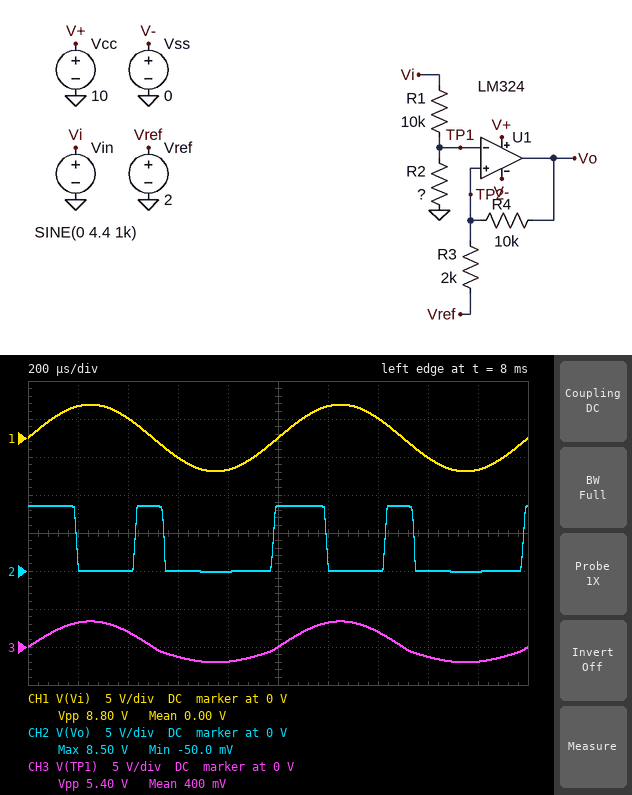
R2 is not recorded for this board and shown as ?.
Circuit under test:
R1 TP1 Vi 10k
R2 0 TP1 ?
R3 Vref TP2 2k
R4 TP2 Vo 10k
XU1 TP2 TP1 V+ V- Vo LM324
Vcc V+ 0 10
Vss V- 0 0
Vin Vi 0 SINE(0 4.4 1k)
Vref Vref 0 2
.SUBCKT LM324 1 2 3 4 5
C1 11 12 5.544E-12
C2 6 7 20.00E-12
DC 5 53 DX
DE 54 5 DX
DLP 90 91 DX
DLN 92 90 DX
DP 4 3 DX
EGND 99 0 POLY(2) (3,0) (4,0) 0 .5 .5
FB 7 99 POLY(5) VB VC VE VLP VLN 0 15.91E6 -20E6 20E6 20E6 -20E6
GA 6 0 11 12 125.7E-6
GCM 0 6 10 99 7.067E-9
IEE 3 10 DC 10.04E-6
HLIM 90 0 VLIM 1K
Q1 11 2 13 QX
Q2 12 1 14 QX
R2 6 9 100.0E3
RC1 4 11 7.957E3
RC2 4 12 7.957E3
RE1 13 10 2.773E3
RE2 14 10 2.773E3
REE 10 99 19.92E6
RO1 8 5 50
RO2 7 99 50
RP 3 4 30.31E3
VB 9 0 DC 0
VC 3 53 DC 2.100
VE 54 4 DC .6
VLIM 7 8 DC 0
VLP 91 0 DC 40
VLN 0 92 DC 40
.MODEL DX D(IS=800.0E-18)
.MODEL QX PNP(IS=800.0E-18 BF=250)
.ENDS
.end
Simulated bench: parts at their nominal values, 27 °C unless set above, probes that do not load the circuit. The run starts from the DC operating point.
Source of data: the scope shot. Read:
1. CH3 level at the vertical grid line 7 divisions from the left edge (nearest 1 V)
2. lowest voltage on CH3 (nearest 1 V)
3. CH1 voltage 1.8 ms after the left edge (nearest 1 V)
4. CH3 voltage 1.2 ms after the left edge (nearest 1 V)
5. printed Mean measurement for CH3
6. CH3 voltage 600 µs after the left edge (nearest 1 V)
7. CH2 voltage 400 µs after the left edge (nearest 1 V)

2 V
-2 V
-4 V
3 V
400 mV
-1 V
0 V
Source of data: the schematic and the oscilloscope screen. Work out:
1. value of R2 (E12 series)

33 kΩ
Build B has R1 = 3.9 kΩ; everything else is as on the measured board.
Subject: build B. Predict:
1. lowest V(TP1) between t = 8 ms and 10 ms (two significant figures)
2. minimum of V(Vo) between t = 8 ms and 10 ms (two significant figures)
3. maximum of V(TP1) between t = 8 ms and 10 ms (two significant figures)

-2.9 V
-82 mV
3.9 V
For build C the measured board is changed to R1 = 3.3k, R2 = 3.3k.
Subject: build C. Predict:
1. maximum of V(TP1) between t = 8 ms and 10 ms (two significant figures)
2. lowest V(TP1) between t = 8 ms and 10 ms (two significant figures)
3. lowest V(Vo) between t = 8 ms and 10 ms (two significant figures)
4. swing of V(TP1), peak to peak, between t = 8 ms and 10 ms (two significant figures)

2.2 V
-1.9 V
-67 mV
4.1 V
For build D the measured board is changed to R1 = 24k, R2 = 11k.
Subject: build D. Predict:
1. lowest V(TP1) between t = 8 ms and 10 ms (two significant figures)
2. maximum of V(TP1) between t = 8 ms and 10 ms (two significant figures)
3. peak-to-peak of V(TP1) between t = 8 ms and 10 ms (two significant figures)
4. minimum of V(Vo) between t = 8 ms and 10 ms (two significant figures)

-980 mV
1.4 V
2.4 V
-33 mV
